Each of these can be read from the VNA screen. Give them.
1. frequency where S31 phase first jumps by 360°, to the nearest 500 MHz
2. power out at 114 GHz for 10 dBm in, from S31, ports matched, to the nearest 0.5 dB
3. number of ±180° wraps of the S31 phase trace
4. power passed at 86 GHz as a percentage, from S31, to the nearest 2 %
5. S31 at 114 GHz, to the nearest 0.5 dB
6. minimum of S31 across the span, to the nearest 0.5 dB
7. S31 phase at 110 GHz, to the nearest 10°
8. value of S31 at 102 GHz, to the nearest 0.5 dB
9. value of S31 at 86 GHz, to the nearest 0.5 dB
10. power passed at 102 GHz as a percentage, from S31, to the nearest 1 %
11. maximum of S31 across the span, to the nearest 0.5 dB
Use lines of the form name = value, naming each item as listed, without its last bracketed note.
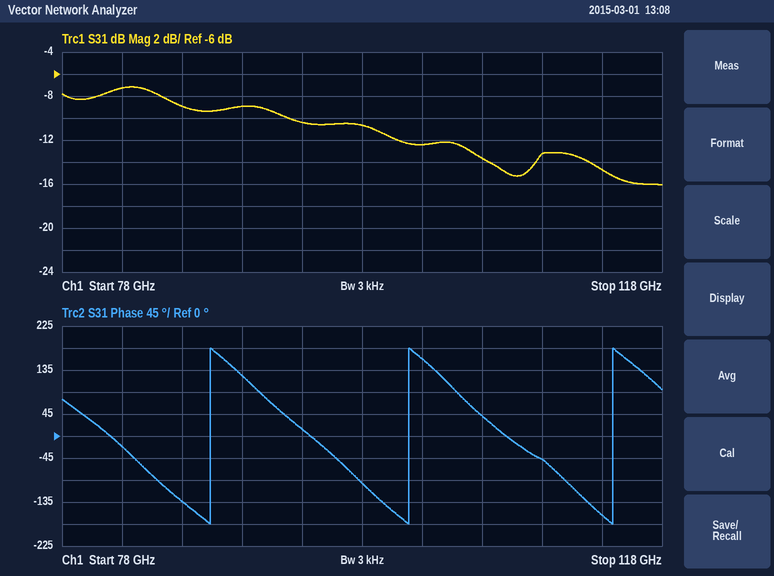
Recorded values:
frequency where S31 phase first jumps by 360°, to the nearest 500 MHz = 88.0 GHz
power out at 114 GHz for 10 dBm in, from S31, ports matched, to the nearest 0.5 dB = -4.5 dBm
number of ±180° wraps of the S31 phase trace = 3
power passed at 86 GHz as a percentage, from S31, to the nearest 2 % = 12 %
S31 at 114 GHz, to the nearest 0.5 dB = -14.5 dB
minimum of S31 across the span, to the nearest 0.5 dB = -16.0 dB
S31 phase at 110 GHz, to the nearest 10° = -50°
value of S31 at 102 GHz, to the nearest 0.5 dB = -12.5 dB
value of S31 at 86 GHz, to the nearest 0.5 dB = -9.0 dB
power passed at 102 GHz as a percentage, from S31, to the nearest 1 % = 6 %
maximum of S31 across the span, to the nearest 0.5 dB = -7.0 dB
